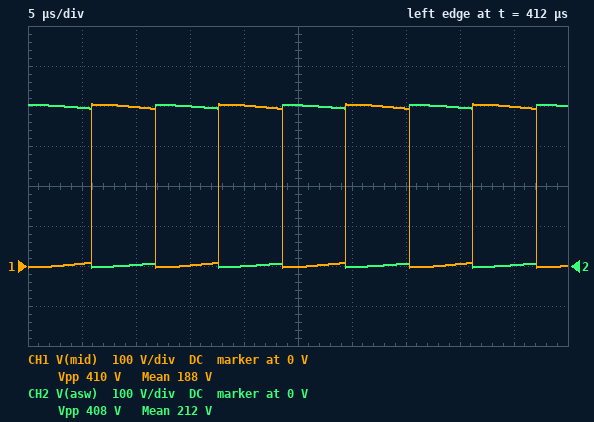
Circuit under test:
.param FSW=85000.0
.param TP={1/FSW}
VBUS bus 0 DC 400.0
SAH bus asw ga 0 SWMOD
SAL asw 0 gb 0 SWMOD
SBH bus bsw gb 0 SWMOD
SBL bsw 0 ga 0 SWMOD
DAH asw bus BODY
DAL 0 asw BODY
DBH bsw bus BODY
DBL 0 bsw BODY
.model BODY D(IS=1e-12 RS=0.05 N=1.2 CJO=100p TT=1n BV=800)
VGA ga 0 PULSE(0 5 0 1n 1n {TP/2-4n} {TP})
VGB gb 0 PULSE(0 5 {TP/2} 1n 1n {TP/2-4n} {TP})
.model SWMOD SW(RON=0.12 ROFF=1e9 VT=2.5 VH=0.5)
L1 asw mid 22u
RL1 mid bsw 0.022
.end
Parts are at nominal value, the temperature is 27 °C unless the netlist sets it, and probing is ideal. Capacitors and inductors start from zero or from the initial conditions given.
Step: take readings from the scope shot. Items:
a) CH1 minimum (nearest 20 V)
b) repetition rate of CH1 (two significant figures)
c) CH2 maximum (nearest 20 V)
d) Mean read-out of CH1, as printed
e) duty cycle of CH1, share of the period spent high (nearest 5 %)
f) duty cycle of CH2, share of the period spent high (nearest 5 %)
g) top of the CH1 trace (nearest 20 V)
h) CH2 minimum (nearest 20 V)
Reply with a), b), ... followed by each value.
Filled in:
a) 0 V
b) 85 kHz
c) 400 V
d) 188 V
e) 50 %
f) 50 %
g) 400 V
h) 0 V
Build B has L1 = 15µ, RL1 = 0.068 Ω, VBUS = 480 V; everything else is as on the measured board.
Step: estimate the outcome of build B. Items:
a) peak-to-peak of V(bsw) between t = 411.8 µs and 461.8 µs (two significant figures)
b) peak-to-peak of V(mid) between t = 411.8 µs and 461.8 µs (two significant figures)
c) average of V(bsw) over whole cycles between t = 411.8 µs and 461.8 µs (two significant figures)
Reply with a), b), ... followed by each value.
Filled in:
a) 490 V
b) 500 V
c) 240 V
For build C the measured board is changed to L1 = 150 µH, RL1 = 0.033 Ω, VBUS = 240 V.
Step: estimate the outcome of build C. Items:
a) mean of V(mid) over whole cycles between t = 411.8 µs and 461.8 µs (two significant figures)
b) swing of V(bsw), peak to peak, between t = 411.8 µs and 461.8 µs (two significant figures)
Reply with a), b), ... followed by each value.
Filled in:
a) 120 V
b) 240 V
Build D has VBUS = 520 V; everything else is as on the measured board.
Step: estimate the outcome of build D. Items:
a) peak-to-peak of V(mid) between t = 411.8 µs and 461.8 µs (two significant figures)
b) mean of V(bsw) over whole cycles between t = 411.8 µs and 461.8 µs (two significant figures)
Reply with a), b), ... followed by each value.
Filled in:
a) 530 V
b) 260 V
